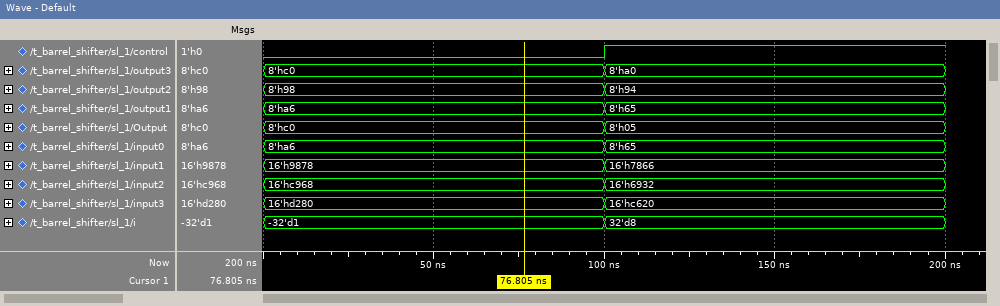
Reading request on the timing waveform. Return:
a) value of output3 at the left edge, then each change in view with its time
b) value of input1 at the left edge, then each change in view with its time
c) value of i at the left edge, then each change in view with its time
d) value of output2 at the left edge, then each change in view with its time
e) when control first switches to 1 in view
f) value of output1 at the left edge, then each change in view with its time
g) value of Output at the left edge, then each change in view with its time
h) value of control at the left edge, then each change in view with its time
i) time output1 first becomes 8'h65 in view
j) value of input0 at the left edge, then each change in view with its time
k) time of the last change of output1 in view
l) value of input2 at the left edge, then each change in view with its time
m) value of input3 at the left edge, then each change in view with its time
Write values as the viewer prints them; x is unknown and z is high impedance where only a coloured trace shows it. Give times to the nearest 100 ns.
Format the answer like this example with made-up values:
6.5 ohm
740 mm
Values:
8'hc0, 8'ha0 at 100 ns
16'h9878, 16'h7866 at 100 ns
-32'd1, 32'd8 at 100 ns
8'h98, 8'h94 at 100 ns
100 ns
8'ha6, 8'h65 at 100 ns
8'hc0, 8'h05 at 100 ns
0, 1 at 100 ns
100 ns
8'ha6, 8'h65 at 100 ns
100 ns
16'hc968, 16'h6932 at 100 ns
16'hd280, 16'hc620 at 100 ns
